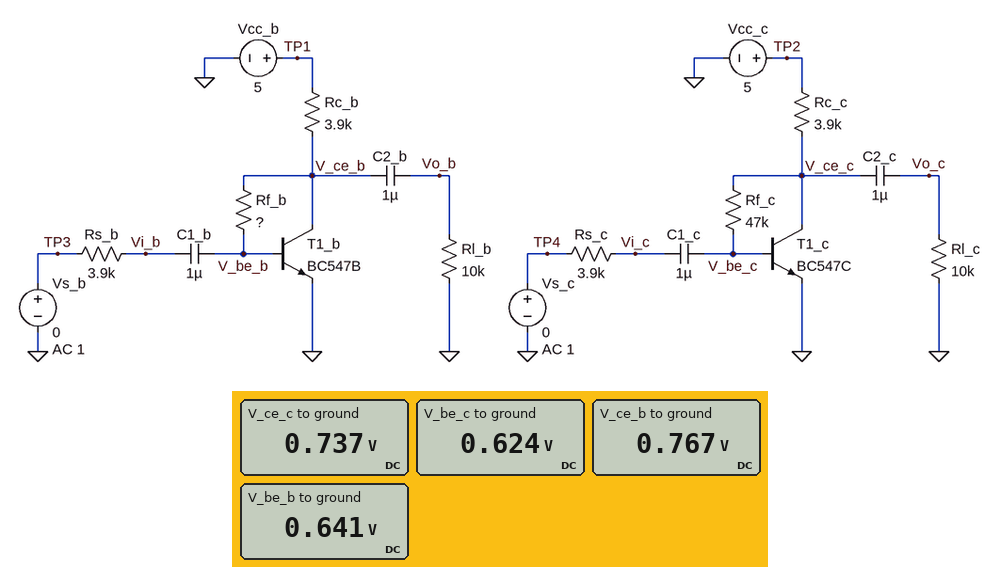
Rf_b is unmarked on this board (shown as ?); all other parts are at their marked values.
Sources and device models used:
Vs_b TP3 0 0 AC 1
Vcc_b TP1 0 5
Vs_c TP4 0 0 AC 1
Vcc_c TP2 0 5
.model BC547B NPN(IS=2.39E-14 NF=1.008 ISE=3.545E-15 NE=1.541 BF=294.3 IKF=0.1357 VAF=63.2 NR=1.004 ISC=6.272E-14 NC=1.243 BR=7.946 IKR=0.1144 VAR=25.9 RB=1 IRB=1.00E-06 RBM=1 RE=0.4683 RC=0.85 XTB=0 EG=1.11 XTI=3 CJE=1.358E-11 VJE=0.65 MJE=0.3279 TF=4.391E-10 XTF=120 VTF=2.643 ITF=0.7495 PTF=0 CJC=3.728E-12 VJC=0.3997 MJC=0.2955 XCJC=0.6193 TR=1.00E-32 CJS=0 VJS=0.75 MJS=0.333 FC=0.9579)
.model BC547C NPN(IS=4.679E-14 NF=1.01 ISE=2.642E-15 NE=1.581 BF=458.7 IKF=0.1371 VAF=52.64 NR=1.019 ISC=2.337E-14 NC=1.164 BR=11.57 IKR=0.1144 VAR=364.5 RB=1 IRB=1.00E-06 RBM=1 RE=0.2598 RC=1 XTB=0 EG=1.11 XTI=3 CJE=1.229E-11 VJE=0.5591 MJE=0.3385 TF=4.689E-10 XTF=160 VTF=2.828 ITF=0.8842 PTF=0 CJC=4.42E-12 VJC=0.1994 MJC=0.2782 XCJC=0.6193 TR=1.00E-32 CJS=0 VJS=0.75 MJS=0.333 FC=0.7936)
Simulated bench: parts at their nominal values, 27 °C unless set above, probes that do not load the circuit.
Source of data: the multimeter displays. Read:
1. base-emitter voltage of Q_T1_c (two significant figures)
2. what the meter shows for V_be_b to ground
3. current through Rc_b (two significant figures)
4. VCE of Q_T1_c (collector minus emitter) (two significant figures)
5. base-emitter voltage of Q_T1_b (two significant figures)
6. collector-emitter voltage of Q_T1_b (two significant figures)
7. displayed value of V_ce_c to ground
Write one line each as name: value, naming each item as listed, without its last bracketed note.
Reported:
base-emitter voltage of Q_T1_c: 620 mV
what the meter shows for V_be_b to ground: 0.641 V
current through Rc_b: 1.1 mA
VCE of Q_T1_c (collector minus emitter): 740 mV
base-emitter voltage of Q_T1_b: 640 mV
collector-emitter voltage of Q_T1_b: 770 mV
displayed value of V_ce_c to ground: 0.737 V
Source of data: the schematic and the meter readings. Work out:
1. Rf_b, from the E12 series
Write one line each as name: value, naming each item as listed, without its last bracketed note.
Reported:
Rf_b, from the E12 series: 33 kΩ
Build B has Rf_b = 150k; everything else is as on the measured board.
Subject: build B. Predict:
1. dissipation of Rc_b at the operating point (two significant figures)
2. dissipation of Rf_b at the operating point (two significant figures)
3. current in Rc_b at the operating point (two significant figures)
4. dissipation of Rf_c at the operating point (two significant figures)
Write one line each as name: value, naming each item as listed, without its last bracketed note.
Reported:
dissipation of Rc_b at the operating point: 3.8 mW
dissipation of Rf_b at the operating point: 1.8 µW
current in Rc_b at the operating point: 990 µA
dissipation of Rf_c at the operating point: 270 nW
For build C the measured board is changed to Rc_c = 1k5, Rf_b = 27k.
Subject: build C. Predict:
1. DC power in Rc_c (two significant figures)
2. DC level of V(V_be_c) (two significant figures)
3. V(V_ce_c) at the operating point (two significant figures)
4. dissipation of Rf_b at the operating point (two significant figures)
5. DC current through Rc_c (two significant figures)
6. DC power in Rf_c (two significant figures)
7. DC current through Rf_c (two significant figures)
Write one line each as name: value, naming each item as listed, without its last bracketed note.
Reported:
DC power in Rc_c: 11 mW
DC level of V(V_be_c): 650 mV
V(V_ce_c) at the operating point: 930 mV
dissipation of Rf_b at the operating point: 400 nW
DC current through Rc_c: 2.7 mA
DC power in Rf_c: 1.7 µW
DC current through Rf_c: 6.0 µA
